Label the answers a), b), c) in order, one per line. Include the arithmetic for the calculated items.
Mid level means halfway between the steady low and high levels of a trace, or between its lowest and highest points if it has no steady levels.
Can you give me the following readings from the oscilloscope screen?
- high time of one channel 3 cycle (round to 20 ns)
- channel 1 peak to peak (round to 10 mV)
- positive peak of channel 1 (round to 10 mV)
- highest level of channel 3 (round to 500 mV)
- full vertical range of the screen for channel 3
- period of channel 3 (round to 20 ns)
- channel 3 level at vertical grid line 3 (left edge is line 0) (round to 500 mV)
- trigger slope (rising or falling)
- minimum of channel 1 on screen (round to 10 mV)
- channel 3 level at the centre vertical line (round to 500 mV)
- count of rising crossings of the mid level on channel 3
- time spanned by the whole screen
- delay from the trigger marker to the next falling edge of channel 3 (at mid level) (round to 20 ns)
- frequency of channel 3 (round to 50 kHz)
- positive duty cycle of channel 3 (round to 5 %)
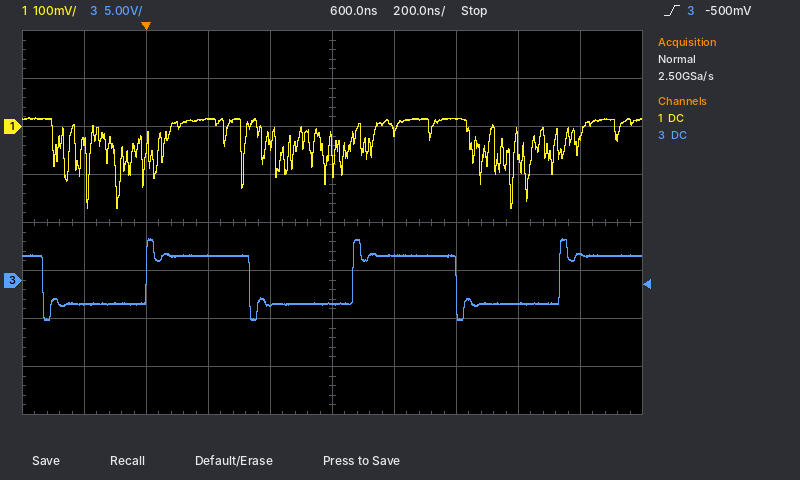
a) 340 ns
b) 20 mV − (-170 mV) = 190 mV
c) 20 mV
d) 4.5 V
e) 40 V
f) 660 ns
g) 2.5 V
h) rising
i) -170 mV
j) -2.5 V
k) 3
l) 2 µs
m) 340 ns
n) 1 / 660 ns ≈ 1.52 MHz, so 1.50 MHz to the nearest 50 kHz
o) 340 ns / 660 ns ≈ 51.5 %, so 50 % to the nearest 5 %
